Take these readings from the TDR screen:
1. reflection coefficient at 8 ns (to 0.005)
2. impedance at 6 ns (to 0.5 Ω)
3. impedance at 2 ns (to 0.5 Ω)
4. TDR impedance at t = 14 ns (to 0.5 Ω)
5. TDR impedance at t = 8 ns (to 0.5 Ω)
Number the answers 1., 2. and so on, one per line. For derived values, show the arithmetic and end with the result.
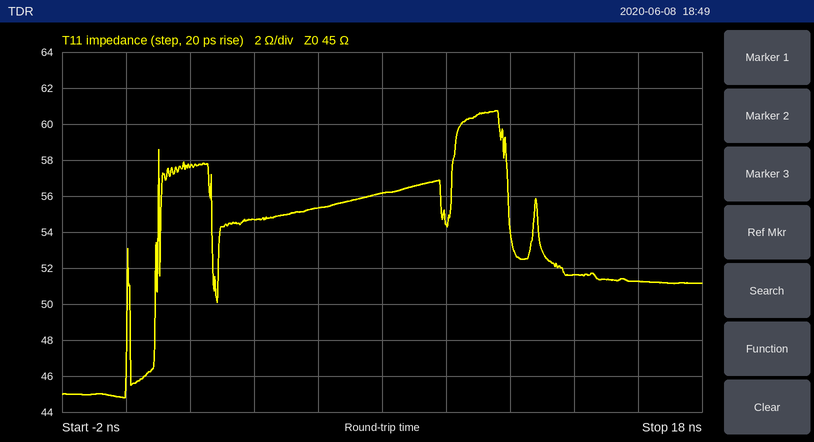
1. (56 − 45)/(56 + 45) ≈ +0.109, so +0.110 to the nearest 0.005
2. 55.5 Ω
3. 57.5 Ω
4. 51.5 Ω
5. 56.0 Ω
